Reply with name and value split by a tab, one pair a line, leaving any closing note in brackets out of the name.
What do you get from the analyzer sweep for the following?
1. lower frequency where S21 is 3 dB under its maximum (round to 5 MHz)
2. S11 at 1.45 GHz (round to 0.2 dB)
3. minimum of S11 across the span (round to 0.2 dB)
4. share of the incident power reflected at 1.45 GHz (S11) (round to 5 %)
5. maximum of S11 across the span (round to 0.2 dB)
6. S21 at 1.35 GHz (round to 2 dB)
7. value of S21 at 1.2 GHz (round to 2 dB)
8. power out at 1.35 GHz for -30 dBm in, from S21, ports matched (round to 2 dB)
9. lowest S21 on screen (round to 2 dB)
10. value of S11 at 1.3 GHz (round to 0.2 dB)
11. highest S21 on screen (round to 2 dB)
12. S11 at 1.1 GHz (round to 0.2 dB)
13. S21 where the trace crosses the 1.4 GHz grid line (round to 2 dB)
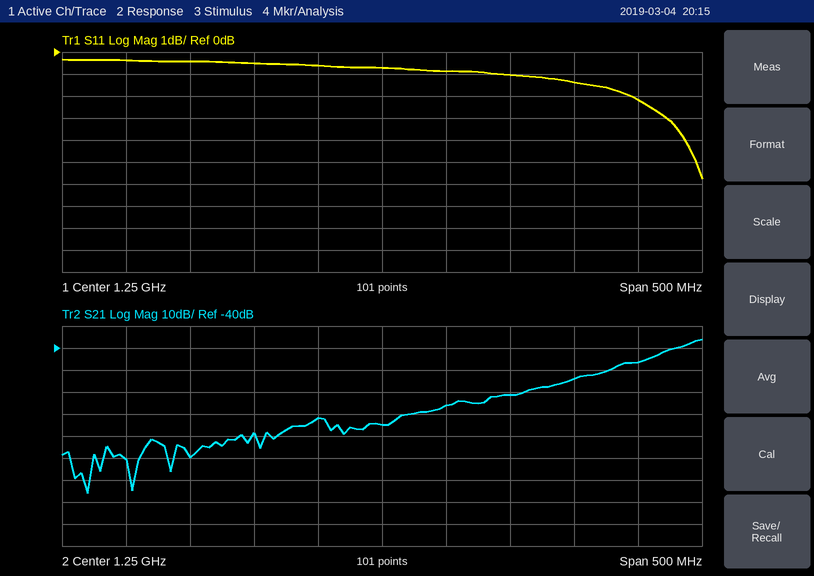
lower frequency where S21 is 3 dB under its maximum	1.485 GHz
S11 at 1.45 GHz	-2.2 dB
minimum of S11 across the span	-5.8 dB
share of the incident power reflected at 1.45 GHz (S11)	60 %
maximum of S11 across the span	-0.4 dB
S21 at 1.35 GHz	-62 dB
value of S21 at 1.2 GHz	-72 dB
power out at 1.35 GHz for -30 dBm in, from S21, ports matched	-92 dBm
lowest S21 on screen	-106 dB
value of S11 at 1.3 GHz	-0.8 dB
highest S21 on screen	-36 dB
S11 at 1.1 GHz	-0.4 dB
S21 where the trace crosses the 1.4 GHz grid line	-54 dB
